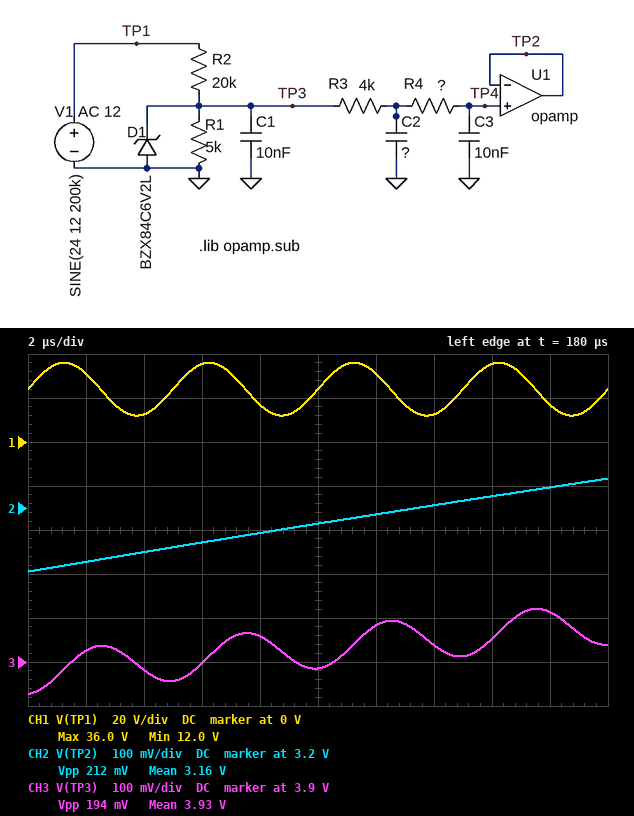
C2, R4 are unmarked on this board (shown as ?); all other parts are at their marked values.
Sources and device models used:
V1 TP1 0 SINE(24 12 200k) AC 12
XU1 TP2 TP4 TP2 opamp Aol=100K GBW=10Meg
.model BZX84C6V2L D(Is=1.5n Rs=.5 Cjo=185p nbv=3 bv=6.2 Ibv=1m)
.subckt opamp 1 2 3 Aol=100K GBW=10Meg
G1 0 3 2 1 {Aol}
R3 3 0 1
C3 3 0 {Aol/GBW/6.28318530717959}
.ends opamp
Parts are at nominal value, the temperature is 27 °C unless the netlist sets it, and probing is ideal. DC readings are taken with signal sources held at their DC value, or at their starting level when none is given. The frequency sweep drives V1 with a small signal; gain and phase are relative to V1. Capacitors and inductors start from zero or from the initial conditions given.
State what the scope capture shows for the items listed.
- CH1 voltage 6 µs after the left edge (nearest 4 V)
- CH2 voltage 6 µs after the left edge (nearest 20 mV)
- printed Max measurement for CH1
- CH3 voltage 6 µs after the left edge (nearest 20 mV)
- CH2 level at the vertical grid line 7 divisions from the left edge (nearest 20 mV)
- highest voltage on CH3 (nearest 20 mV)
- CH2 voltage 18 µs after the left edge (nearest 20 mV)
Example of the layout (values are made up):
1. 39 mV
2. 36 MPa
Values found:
1. 36 V
2. 3.12 V
3. 36.0 V
4. 3.90 V
5. 3.20 V
6. 4.02 V
7. 3.24 V
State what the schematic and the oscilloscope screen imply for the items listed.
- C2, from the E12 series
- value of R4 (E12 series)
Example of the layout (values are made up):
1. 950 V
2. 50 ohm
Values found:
1. 5.6 nF
2. 1.2 kΩ
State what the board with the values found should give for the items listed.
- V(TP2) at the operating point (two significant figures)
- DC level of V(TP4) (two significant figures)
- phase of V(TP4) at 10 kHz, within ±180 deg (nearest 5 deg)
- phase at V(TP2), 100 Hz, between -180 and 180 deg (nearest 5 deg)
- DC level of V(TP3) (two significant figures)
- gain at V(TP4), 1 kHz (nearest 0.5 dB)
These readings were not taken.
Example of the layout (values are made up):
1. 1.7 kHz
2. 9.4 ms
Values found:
1. 4.8 V
2. 4.8 V
3. -145 deg
4. -5 deg
5. 4.8 V
6. -17.0 dB
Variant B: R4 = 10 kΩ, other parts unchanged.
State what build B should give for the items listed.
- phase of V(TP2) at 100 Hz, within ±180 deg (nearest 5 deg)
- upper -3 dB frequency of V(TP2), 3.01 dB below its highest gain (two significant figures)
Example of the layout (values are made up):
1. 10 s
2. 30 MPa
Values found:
1. -10 deg
2. 710 Hz
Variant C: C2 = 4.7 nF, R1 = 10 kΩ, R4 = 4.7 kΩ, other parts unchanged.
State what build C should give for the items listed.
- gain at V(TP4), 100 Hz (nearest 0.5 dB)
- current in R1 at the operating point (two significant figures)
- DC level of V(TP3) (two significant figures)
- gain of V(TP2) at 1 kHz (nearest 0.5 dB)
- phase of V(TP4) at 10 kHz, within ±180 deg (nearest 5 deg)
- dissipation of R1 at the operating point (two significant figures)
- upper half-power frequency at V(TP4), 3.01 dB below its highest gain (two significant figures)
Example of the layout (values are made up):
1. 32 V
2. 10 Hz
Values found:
1. -37.5 dB
2. 610 µA
3. 6.1 V
4. -39.0 dB
5. -120 deg
6. 3.7 mW
7. 1.6 kHz
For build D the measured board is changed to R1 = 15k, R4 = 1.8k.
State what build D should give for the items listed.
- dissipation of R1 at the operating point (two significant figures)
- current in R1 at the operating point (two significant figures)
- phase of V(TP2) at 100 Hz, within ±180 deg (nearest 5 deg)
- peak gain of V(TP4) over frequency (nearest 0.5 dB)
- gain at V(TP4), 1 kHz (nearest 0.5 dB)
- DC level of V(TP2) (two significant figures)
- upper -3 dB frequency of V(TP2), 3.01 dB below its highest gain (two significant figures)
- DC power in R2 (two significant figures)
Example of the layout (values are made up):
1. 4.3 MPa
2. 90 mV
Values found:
1. 2.5 mW
2. 410 µA
3. -5 deg
4. -42.0 dB
5. -43.0 dB
6. 6.1 V
7. 2.0 kHz
8. 16 mW
